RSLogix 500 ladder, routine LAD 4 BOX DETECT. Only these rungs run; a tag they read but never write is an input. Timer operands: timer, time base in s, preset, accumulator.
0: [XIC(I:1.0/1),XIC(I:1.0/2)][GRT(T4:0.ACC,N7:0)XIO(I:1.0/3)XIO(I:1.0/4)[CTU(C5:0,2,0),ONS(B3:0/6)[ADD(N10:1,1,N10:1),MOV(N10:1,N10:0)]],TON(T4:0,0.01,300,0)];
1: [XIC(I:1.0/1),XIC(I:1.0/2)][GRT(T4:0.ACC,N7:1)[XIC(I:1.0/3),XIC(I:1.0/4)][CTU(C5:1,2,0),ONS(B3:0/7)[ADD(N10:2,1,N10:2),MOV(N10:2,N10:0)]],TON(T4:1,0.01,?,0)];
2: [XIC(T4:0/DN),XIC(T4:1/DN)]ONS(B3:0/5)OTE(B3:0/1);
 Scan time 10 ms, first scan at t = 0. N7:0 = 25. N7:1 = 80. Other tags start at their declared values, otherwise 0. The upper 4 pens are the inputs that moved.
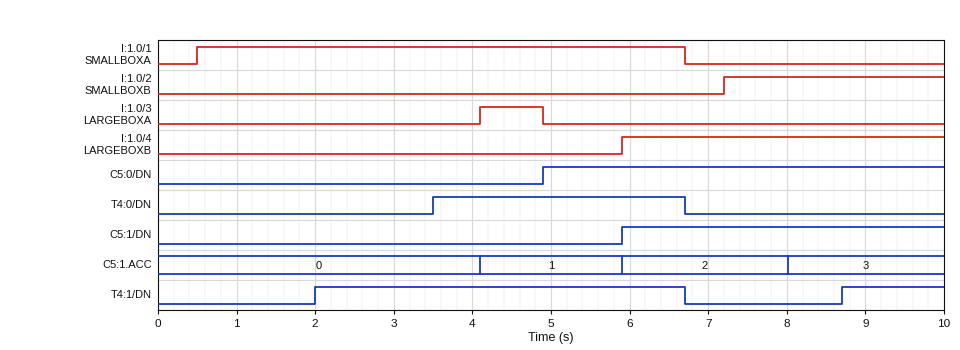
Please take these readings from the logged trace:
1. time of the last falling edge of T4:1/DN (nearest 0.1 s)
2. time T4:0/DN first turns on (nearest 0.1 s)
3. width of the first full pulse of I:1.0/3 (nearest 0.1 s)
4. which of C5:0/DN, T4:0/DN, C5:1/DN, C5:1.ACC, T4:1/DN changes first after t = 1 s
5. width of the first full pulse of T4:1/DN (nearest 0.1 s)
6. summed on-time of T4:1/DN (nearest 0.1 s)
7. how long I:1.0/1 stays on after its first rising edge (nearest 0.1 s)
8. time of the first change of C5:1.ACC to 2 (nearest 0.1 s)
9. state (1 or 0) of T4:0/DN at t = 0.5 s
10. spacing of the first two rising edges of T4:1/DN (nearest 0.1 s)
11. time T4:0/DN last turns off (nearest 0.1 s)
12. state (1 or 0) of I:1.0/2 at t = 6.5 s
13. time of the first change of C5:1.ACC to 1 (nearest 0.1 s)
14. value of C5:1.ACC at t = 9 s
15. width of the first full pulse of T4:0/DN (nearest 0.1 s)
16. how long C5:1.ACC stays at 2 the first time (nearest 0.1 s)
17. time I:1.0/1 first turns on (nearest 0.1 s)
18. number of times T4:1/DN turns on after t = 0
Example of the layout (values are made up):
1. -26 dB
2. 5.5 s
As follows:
1. 6.7 s
2. 3.5 s
3. 0.8 s
4. T4:1/DN
5. 4.7 s
6. 6.0 s
7. 6.2 s
8. 5.9 s
9. 0
10. 6.7 s
11. 6.7 s
12. 0
13. 4.1 s
14. 3
15. 3.2 s
16. 2.1 s
17. 0.5 s
18. 2
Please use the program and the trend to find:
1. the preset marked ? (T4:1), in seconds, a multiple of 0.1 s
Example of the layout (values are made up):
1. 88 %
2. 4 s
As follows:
1. 1.5 s
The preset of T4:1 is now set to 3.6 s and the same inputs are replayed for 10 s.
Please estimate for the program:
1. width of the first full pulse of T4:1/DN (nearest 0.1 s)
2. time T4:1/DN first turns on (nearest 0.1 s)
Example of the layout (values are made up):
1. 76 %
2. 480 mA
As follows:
1. 2.6 s
2. 4.1 s
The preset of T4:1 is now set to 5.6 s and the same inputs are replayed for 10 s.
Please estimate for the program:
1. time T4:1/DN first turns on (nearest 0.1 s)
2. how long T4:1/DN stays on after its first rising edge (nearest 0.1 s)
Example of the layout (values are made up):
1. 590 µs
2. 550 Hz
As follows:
1. 6.1 s
2. 0.6 s
